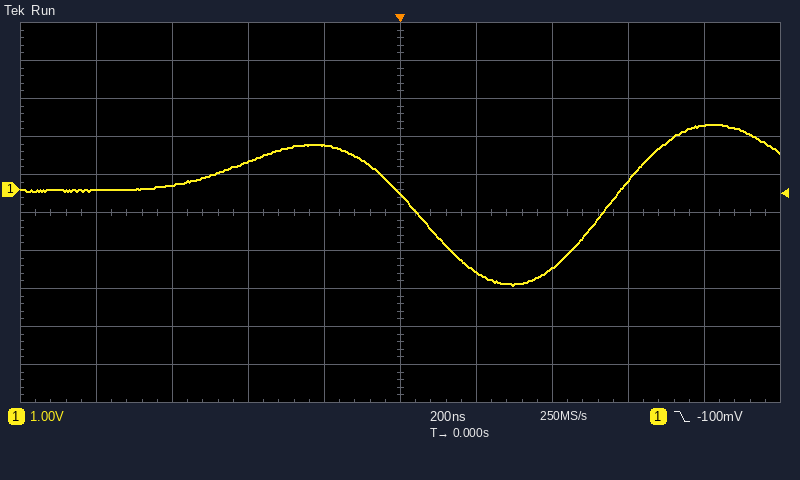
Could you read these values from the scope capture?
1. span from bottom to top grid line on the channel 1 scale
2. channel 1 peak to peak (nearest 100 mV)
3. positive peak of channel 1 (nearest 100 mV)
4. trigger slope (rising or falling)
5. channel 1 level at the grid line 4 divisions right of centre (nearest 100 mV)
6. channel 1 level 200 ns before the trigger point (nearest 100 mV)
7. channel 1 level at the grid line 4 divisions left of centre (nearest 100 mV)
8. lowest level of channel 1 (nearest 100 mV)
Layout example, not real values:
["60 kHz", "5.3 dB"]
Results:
["10 V", "4.2 V", "1.7 V", "falling", "1.7 V", "1.2 V", "0.0 V", "-2.5 V"]
